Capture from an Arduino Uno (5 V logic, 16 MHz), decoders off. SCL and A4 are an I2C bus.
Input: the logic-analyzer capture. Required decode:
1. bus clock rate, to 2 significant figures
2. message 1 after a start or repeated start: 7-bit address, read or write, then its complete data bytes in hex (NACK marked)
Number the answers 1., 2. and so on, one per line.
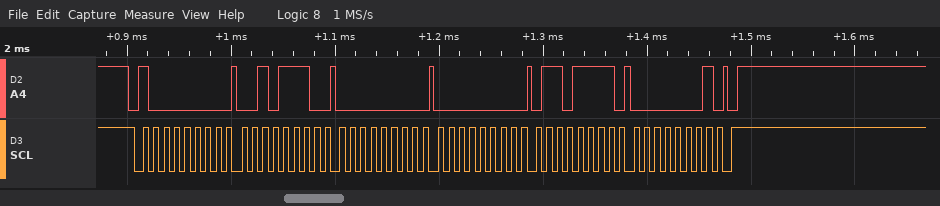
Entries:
1. 100 kHz
2. 0x40 write: 2E 00 00 6F 01
